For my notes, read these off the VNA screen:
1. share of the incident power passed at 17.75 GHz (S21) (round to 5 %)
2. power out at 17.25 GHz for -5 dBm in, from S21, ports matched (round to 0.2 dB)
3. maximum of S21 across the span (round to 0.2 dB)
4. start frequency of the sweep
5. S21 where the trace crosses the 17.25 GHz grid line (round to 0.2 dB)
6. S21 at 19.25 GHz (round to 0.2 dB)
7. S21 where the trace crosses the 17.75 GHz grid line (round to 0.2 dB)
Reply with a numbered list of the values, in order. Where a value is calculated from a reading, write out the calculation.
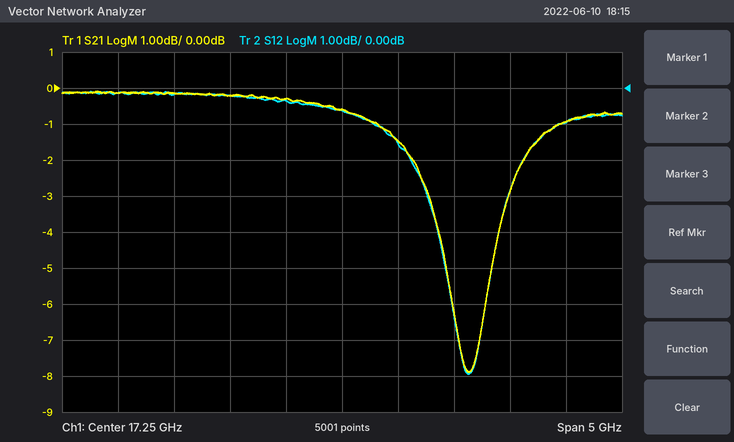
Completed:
1. 10^(-1.4/10) ≈ 72.4 %, so 70 % to the nearest 5 %
2. -5 dBm + (-0.6 dB) = -5.6 dBm
3. 0.0 dB
4. 14.75 GHz
5. -0.6 dB
6. -1.0 dB
7. -1.4 dB
